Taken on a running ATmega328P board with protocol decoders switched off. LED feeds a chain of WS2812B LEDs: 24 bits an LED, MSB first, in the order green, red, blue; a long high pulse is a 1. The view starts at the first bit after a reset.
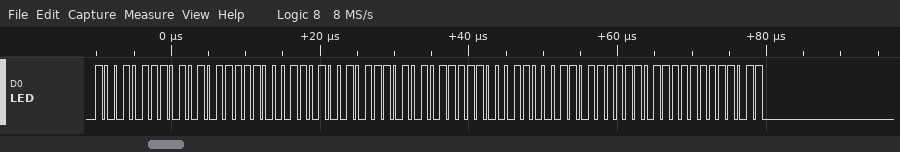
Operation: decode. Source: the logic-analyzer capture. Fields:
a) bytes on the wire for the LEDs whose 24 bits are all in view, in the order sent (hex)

97 57 C6 97 57 C6 37 EF FB
